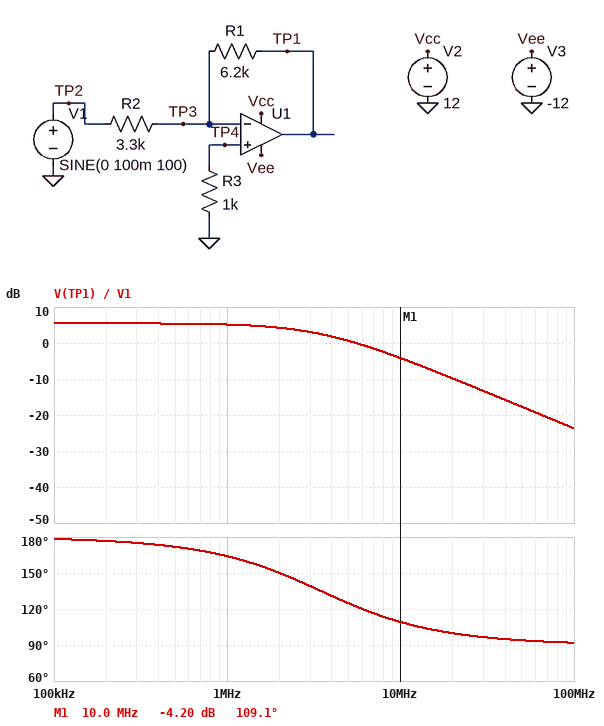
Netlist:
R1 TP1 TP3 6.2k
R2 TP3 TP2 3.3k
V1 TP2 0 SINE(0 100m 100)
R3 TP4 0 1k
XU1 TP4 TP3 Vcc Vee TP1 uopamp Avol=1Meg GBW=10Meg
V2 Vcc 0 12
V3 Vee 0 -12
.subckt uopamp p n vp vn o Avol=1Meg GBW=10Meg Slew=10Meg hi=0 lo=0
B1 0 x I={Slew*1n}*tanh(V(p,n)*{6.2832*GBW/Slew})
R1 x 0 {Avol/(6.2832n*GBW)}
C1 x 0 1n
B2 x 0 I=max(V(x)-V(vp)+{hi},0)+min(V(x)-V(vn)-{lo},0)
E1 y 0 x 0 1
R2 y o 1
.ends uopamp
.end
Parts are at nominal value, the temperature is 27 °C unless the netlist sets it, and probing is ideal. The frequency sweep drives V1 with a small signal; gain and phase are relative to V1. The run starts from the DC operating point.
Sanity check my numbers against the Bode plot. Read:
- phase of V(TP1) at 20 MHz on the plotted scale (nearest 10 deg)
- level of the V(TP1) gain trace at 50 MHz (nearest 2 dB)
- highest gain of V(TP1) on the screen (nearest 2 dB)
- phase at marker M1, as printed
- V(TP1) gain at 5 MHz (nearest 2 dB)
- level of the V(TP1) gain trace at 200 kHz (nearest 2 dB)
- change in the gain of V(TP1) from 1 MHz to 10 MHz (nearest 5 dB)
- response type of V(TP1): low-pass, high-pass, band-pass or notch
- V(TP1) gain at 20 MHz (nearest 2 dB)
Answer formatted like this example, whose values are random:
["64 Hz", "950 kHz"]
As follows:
["100 deg", "-18 dB", "6 dB", "109.1 deg", "0 dB", "6 dB", "-10 dB", "low-pass", "-10 dB"]
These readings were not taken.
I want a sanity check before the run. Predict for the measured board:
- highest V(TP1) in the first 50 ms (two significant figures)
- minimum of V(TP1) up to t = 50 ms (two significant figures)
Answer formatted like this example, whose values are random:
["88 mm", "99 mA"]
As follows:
["190 mV", "-190 mV"]
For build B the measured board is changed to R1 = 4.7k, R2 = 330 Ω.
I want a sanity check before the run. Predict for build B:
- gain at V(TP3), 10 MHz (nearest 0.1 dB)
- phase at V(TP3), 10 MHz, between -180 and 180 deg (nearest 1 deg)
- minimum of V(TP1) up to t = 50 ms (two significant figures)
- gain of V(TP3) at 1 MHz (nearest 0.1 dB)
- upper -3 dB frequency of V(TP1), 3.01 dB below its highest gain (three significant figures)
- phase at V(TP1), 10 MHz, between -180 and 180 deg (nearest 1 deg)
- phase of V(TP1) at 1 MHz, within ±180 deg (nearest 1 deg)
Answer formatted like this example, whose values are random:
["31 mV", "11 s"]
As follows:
["-0.6 dB", "4 deg", "-1.4 V", "-2.1 dB", "656 kHz", "94 deg", "123 deg"]
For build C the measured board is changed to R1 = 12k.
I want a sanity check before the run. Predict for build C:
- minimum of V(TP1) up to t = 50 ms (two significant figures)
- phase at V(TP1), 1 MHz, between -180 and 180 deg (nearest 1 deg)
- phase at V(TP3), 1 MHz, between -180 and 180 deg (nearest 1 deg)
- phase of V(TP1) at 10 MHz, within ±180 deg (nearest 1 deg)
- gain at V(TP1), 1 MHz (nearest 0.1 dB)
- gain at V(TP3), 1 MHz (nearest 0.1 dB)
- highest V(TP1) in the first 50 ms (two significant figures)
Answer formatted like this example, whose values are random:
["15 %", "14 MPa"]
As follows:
["-360 mV", "155 deg", "65 deg", "102 deg", "10.4 dB", "-9.6 dB", "360 mV"]
